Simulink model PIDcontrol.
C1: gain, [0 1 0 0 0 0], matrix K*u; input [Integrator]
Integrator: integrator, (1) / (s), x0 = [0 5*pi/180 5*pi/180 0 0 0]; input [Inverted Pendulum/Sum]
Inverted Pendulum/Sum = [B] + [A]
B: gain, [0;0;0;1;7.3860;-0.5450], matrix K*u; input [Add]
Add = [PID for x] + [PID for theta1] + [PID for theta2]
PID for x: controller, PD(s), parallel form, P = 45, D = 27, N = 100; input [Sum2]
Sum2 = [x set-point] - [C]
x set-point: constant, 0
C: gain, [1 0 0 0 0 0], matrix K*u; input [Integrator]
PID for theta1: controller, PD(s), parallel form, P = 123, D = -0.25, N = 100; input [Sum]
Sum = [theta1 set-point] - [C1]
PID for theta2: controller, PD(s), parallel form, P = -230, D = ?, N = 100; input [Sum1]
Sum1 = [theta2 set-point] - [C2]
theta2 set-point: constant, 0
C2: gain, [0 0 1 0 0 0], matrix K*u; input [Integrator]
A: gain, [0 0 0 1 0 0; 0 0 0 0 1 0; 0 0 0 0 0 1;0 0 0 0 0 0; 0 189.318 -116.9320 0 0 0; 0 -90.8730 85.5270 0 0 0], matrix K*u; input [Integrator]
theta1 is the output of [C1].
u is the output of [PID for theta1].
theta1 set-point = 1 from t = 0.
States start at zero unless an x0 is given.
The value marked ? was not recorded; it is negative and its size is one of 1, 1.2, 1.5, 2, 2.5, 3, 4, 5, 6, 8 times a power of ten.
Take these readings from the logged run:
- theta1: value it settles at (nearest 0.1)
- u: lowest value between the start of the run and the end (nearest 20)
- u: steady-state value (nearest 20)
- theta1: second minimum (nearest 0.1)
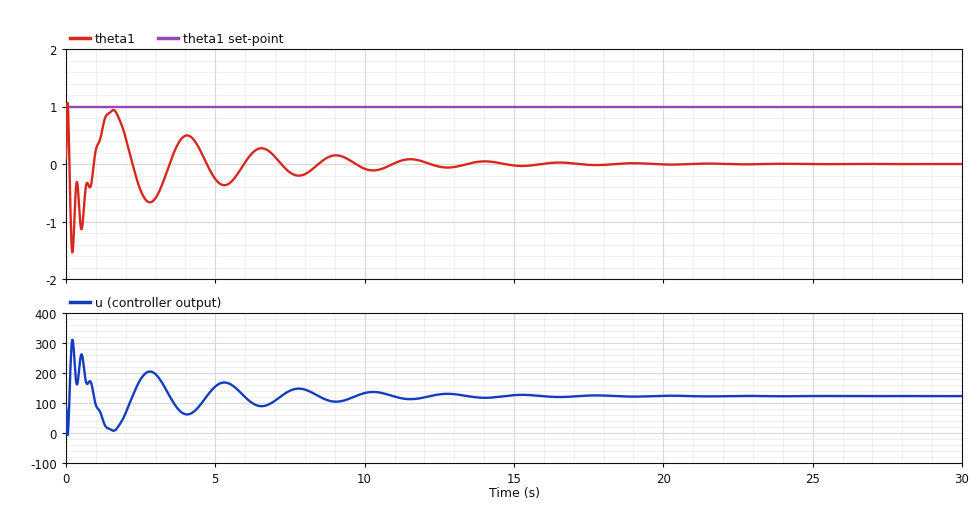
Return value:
0.0
0
120
-1.1
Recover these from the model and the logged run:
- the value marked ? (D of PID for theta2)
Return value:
-50
